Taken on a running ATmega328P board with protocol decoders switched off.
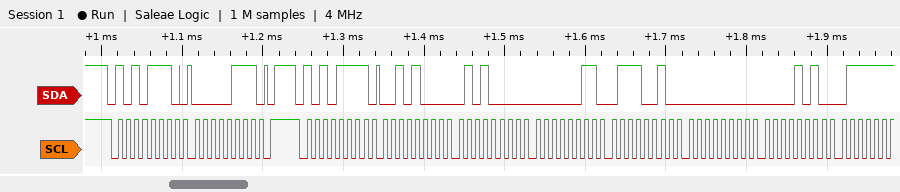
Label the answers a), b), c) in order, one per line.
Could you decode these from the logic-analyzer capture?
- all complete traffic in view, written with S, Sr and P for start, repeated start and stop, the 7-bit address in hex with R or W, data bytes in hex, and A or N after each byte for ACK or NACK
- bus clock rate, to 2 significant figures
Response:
a) S 57W A 07 A P S 57R A 28 A 50 A 03 A 72 A 00 A 0A A
b) 100 kHz
